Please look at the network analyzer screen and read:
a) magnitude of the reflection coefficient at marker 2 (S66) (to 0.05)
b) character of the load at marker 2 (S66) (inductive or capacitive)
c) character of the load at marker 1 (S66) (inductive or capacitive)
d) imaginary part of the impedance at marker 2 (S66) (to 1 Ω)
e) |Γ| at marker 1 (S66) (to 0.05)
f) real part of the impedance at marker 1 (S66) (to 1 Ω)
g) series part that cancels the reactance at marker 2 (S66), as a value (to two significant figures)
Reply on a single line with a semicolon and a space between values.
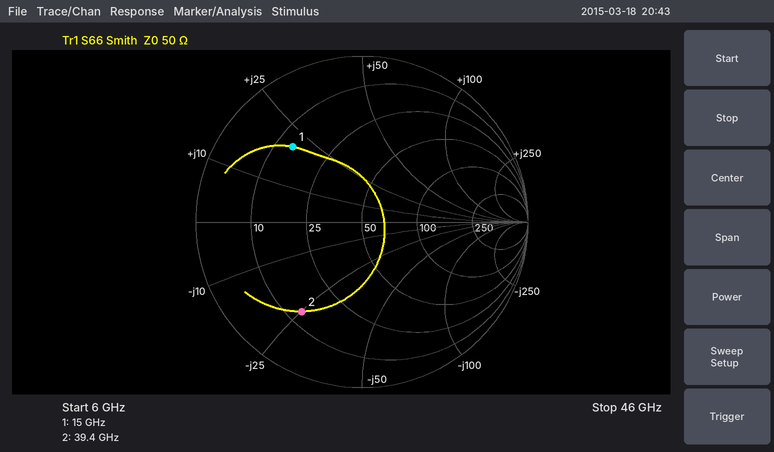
0.65; capacitive; inductive; -25 Ω; 0.60; 14 Ω; 100 pH
